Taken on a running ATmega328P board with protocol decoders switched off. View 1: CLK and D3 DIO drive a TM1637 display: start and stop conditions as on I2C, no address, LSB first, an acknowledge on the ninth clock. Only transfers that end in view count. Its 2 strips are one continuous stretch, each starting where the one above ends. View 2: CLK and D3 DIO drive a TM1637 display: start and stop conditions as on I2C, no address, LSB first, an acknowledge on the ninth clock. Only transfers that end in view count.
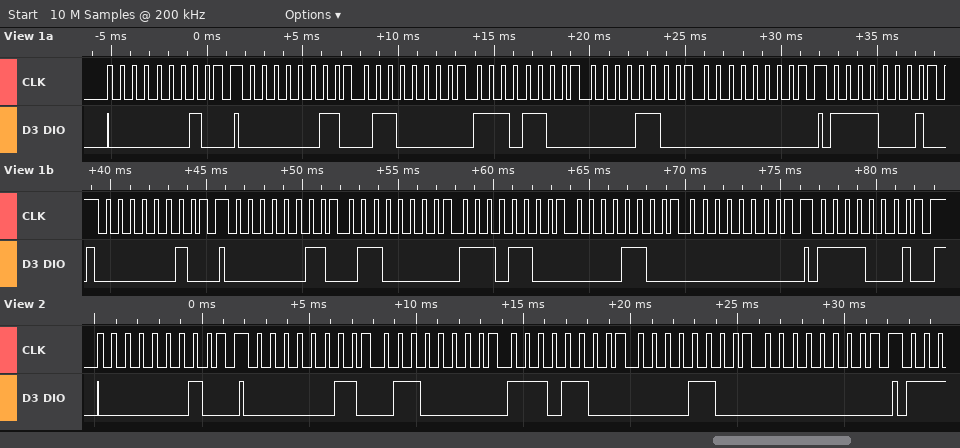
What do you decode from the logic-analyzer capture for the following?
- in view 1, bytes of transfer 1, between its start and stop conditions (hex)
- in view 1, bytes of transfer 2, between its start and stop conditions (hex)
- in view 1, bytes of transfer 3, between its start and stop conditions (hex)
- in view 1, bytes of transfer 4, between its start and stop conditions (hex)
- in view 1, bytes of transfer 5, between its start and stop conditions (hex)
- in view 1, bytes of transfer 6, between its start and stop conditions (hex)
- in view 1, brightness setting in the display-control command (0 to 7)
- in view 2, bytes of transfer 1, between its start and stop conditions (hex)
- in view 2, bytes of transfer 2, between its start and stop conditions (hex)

40
C0 06 37 30 00
8F
40
C0 06 37 30 00
8F
7
40
C0 06 37 30 00
